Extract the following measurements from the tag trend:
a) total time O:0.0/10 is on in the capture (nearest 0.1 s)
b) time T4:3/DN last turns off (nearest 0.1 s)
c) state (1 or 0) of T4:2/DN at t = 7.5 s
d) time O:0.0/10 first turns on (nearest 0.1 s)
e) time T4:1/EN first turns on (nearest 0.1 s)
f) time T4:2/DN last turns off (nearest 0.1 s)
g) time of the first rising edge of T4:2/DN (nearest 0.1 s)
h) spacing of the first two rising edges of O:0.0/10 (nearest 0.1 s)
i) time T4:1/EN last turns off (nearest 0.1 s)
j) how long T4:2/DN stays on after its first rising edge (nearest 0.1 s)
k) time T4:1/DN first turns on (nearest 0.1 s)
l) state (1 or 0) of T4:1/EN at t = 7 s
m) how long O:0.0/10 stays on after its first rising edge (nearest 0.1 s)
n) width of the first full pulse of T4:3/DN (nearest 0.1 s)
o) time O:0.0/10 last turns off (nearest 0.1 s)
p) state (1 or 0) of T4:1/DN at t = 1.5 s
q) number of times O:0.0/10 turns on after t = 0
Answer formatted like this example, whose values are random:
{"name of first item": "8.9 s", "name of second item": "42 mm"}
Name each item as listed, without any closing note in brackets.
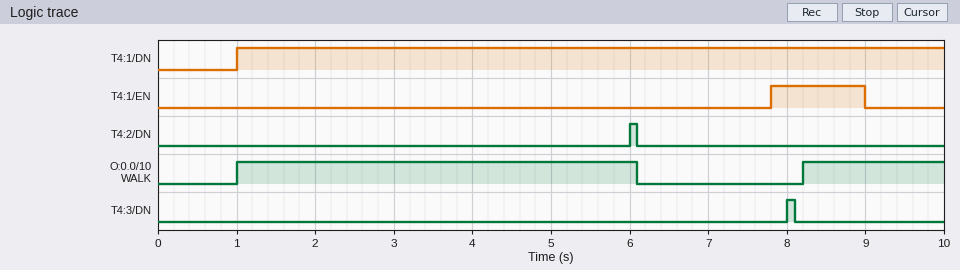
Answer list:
{"total time O:0.0/10 is on in the capture": "6.9 s", "time T4:3/DN last turns off": "8.1 s", "state (1 or 0) of T4:2/DN at t = 7.5 s": "0", "time O:0.0/10 first turns on": "1.0 s", "time T4:1/EN first turns on": "7.8 s", "time T4:2/DN last turns off": "6.1 s", "time of the first rising edge of T4:2/DN": "6.0 s", "spacing of the first two rising edges of O:0.0/10": "7.2 s", "time T4:1/EN last turns off": "9.0 s", "how long T4:2/DN stays on after its first rising edge": "0.1 s", "time T4:1/DN first turns on": "1.0 s", "state (1 or 0) of T4:1/EN at t = 7 s": "0", "how long O:0.0/10 stays on after its first rising edge": "5.1 s", "width of the first full pulse of T4:3/DN": "0.1 s", "time O:0.0/10 last turns off": "6.1 s", "state (1 or 0) of T4:1/DN at t = 1.5 s": "1", "number of times O:0.0/10 turns on after t = 0": "2"}
